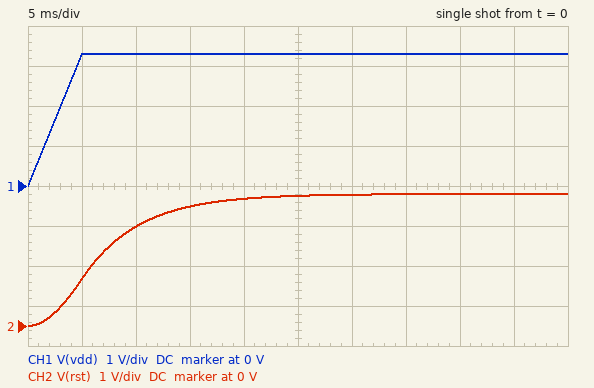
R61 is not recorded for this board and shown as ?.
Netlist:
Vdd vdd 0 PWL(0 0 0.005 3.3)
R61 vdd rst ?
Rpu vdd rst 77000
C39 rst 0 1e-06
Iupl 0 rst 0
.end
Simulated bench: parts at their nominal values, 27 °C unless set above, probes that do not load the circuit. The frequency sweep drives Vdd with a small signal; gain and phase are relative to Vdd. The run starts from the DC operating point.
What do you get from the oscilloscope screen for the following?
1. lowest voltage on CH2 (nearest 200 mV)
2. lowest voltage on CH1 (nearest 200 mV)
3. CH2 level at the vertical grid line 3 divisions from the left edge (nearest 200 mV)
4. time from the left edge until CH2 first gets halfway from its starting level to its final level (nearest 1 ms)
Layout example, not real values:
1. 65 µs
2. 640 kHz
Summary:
1. 0 V
2. 0 V
3. 3.0 V
4. 6 ms
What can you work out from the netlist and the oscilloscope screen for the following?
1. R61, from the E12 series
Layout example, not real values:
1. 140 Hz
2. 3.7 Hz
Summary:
1. 5.6 kΩ
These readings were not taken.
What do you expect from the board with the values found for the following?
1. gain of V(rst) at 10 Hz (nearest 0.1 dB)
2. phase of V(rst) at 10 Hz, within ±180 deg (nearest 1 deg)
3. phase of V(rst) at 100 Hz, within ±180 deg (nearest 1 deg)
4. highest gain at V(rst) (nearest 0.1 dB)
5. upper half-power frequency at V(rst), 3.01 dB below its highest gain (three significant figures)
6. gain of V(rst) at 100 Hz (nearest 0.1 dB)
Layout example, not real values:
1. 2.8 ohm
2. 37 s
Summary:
1. -0.4 dB
2. -18 deg
3. -73 deg
4. 0 dB
5. 30.5 Hz
6. -10.7 dB
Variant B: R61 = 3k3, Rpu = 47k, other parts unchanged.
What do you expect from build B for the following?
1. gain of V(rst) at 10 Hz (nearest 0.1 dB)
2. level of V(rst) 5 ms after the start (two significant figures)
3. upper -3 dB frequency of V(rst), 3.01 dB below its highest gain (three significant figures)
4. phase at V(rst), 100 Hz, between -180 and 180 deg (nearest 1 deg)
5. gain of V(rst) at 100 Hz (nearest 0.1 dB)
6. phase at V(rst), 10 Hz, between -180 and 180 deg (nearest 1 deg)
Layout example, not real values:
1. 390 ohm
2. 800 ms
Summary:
1. -0.2 dB
2. 1.7 V
3. 51.6 Hz
4. -63 deg
5. -6.8 dB
6. -11 deg
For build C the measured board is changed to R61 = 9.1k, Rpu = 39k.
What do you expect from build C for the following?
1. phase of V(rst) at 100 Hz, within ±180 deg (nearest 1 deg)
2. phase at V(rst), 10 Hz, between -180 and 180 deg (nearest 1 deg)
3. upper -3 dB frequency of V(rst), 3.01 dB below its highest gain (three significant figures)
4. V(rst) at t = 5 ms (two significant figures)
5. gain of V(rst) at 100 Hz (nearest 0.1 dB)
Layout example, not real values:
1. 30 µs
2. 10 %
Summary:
1. -78 deg
2. -25 deg
3. 21.6 Hz
4. 900 mV
5. -13.5 dB
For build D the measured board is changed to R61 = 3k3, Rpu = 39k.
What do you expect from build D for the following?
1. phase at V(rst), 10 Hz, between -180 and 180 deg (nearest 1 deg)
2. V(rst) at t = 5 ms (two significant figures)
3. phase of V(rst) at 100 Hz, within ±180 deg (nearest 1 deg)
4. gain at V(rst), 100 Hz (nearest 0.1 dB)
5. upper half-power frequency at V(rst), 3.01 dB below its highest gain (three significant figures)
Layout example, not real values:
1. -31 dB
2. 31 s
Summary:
1. -11 deg
2. 1.7 V
3. -62 deg
4. -6.7 dB
5. 52.3 Hz
